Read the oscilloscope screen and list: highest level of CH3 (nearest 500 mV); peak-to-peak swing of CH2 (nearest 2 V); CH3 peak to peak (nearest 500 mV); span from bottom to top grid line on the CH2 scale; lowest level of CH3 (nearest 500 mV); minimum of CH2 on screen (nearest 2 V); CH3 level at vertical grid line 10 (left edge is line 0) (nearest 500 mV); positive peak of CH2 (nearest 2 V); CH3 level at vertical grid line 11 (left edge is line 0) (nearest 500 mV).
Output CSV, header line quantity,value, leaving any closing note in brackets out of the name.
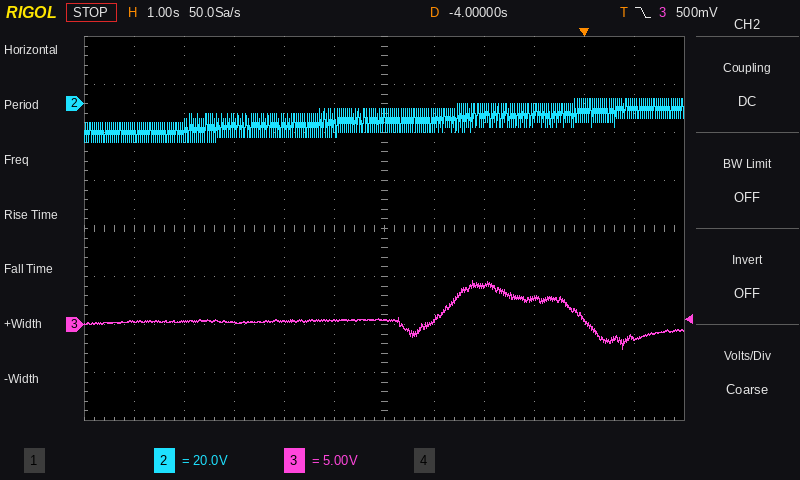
quantity,value
highest level of CH3,4.5 V
peak-to-peak swing of CH2,18 V
CH3 peak to peak,7.0 V
span from bottom to top grid line on the CH2 scale,160 V
lowest level of CH3,-2.5 V
minimum of CH2 on screen,-16 V
CH3 level at vertical grid line 10 (left edge is line 0),500 mV
positive peak of CH2,2 V
CH3 level at vertical grid line 11 (left edge is line 0),-1.5 V
